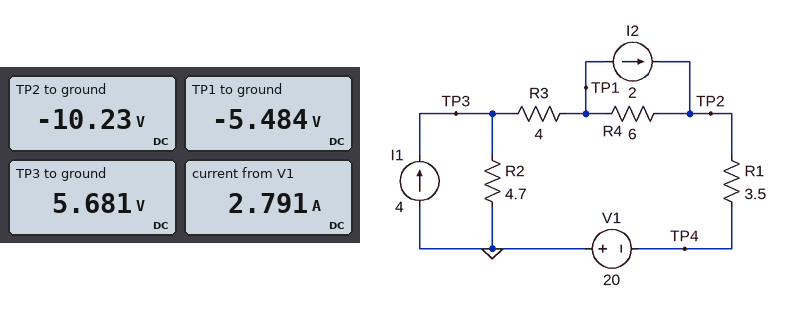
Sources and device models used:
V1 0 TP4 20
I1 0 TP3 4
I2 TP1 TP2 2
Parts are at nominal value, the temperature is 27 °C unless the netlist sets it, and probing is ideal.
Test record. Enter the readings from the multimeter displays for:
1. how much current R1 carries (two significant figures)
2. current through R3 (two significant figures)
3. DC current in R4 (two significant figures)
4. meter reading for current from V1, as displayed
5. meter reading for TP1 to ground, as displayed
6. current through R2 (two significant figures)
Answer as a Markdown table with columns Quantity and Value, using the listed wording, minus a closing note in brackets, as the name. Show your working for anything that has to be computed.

| Quantity | Value |
|---|---|
| how much current R1 carries | (-10.23 V - (-20 V)) / 3.5 Ω = 2.8 A |
| current through R3 | (5.681 V - (-5.484 V)) / 4 Ω = 2.8 A |
| DC current in R4 | (-5.484 V - (-10.23 V)) / 6 Ω = 790 mA |
| meter reading for current from V1, as displayed | 2.791 A |
| meter reading for TP1 to ground, as displayed | -5.484 V |
| current through R2 | (5.681 V) / 4.7 Ω = 1.2 A |
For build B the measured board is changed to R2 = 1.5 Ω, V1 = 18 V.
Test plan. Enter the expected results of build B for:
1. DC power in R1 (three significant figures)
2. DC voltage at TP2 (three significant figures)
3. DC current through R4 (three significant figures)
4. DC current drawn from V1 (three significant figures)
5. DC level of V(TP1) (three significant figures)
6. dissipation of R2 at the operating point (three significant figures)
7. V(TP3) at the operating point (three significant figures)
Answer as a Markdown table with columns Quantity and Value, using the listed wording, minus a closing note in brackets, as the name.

| Quantity | Value |
|---|---|
| DC power in R1 | 20.2 W |
| DC voltage at TP2 | -9.60 V |
| DC current through R4 | 400 mA |
| DC current drawn from V1 | 2.40 A |
| DC level of V(TP1) | -7.20 V |
| dissipation of R2 at the operating point | 3.84 W |
| V(TP3) at the operating point | 2.40 V |
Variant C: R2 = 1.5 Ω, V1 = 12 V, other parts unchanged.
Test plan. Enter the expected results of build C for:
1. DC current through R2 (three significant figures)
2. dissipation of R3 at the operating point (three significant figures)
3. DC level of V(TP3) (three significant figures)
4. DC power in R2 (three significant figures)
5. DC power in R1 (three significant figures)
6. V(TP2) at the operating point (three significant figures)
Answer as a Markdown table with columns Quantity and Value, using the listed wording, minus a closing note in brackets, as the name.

| Quantity | Value |
|---|---|
| DC current through R2 | 2.00 A |
| dissipation of R3 at the operating point | 16.0 W |
| DC level of V(TP3) | 3.00 V |
| DC power in R2 | 6.00 W |
| DC power in R1 | 14.0 W |
| V(TP2) at the operating point | -5.00 V |
